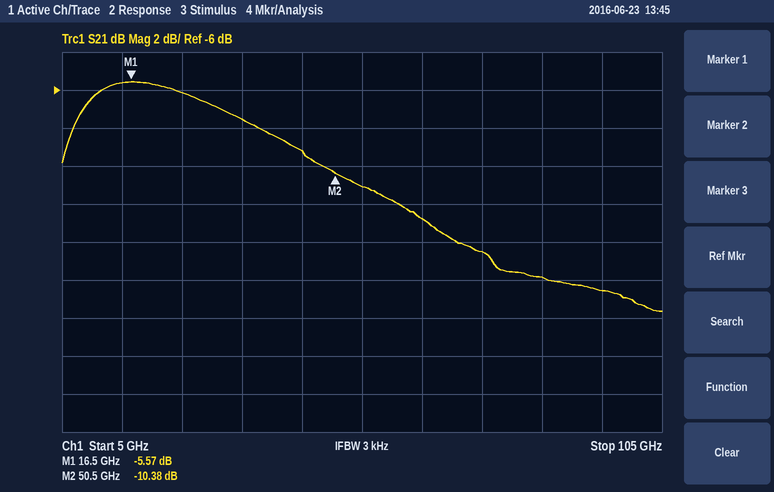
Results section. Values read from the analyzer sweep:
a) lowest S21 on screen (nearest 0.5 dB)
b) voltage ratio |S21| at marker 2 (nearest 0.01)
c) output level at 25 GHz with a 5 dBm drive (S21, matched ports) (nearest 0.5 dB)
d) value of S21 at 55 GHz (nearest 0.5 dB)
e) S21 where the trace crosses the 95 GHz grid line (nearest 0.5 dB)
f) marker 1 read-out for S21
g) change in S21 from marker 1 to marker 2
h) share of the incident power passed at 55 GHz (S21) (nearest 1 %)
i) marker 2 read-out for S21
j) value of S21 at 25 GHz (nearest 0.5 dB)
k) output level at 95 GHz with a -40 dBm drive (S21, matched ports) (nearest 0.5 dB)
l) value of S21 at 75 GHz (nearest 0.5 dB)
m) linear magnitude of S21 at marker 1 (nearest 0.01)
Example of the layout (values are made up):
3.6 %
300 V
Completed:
-17.5 dB
0.30
-1.0 dBm
-11.0 dB
-16.5 dB
-5.57 dB
-4.81 dB
8 %
-10.38 dB
-6.0 dB
-56.5 dBm
-14.5 dB
0.53
